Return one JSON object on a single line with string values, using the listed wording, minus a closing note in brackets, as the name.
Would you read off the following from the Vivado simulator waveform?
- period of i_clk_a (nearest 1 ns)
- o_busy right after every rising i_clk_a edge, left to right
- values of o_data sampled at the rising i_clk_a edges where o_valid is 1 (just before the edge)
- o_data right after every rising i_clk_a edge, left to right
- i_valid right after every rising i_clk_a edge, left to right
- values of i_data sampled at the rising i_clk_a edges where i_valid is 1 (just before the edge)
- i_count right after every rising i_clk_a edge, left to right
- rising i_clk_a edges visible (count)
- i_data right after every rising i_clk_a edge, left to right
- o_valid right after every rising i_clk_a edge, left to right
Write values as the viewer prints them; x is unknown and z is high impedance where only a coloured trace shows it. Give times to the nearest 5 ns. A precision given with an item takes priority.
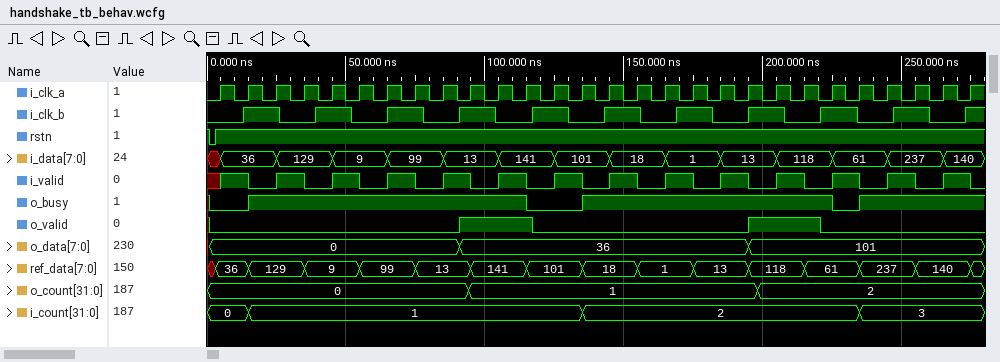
{"period of i_clk_a": "10 ns", "o_busy right after every rising i_clk_a edge, left to right": "0 1 1 1 1 1 1 1 1 1 1 0 0 1 1 1 1 1 1 1 1 1 0 1 1 1 1 1", "values of o_data sampled at the rising i_clk_a edges where o_valid is 1": "36, 36, 36, 101, 101", "o_data right after every rising i_clk_a edge, left to right": "0, 0, 0, 0, 0, 0, 0, 0, 0, 36, 36, 36, 36, 36, 36, 36, 36, 36, 36, 101, 101, 101, 101, 101, 101, 101, 101, 101", "i_valid right after every rising i_clk_a edge, left to right": "1 0 1 0 1 0 1 0 1 0 1 0 1 0 1 0 1 0 1 0 1 0 1 0 1 0 1 0", "values of i_data sampled at the rising i_clk_a edges where i_valid is 1": "36, 129, 9, 99, 13, 141, 101, 18, 1, 13, 118, 61, 237, 140", "i_count right after every rising i_clk_a edge, left to right": "0, 1, 1, 1, 1, 1, 1, 1, 1, 1, 1, 1, 1, 2, 2, 2, 2, 2, 2, 2, 2, 2, 2, 3, 3, 3, 3, 3", "rising i_clk_a edges visible": "28", "i_data right after every rising i_clk_a edge, left to right": "36, 36, 129, 129, 9, 9, 99, 99, 13, 13, 141, 141, 101, 101, 18, 18, 1, 1, 13, 13, 118, 118, 61, 61, 237, 237, 140, 140", "o_valid right after every rising i_clk_a edge, left to right": "0 0 0 0 0 0 0 0 0 1 1 1 0 0 0 0 0 0 0 1 1 1 0 0 0 0 0 0"}
